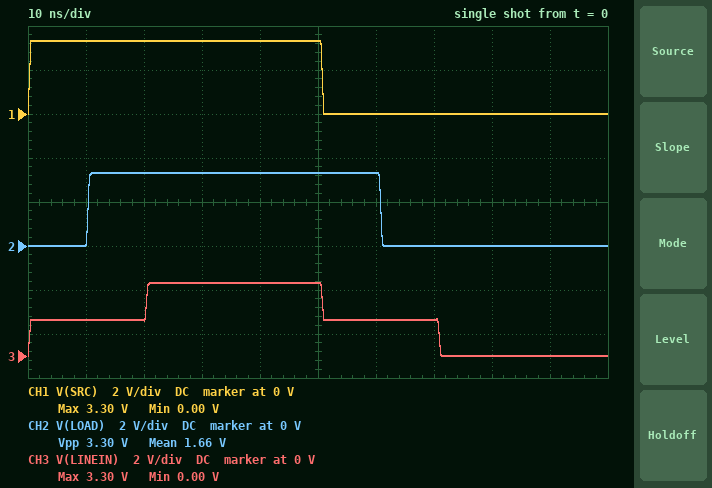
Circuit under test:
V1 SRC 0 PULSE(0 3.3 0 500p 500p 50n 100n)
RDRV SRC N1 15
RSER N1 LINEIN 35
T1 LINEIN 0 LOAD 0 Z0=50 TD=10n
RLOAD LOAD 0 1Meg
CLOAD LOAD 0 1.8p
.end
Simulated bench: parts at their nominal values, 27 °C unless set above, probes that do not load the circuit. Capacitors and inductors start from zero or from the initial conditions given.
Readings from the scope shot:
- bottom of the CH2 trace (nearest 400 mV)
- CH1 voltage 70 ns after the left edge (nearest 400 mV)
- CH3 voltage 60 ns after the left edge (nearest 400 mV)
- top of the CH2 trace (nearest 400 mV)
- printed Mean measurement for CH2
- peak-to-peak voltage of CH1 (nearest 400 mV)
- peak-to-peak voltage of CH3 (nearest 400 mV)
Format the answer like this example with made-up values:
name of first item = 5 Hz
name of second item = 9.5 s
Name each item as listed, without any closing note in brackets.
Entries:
bottom of the CH2 trace = 0 V
CH1 voltage 70 ns after the left edge = 0 V
CH3 voltage 60 ns after the left edge = 1.6 V
top of the CH2 trace = 3.2 V
printed Mean measurement for CH2 = 1.66 V
peak-to-peak voltage of CH1 = 3.2 V
peak-to-peak voltage of CH3 = 3.2 V
